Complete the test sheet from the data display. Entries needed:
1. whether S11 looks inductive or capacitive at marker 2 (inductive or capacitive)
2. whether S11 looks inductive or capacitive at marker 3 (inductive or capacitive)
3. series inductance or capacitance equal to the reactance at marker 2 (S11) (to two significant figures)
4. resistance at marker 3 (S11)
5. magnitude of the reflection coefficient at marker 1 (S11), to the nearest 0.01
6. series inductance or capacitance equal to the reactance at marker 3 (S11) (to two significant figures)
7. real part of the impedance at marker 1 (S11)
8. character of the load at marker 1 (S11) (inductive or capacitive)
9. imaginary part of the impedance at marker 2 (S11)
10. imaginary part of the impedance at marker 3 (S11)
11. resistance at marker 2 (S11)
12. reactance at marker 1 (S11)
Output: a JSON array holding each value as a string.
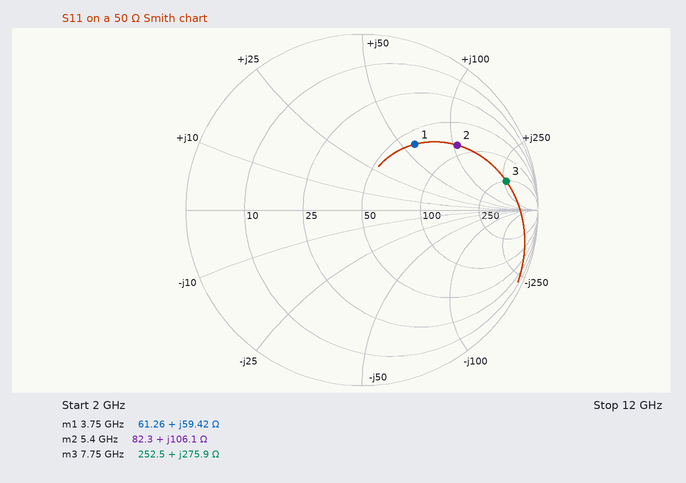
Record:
["inductive", "inductive", "3.1 nH", "252.5 Ω", "0.48", "5.7 nH", "61.26 Ω", "inductive", "+106.1 Ω", "+275.9 Ω", "82.3 Ω", "+59.42 Ω"]
